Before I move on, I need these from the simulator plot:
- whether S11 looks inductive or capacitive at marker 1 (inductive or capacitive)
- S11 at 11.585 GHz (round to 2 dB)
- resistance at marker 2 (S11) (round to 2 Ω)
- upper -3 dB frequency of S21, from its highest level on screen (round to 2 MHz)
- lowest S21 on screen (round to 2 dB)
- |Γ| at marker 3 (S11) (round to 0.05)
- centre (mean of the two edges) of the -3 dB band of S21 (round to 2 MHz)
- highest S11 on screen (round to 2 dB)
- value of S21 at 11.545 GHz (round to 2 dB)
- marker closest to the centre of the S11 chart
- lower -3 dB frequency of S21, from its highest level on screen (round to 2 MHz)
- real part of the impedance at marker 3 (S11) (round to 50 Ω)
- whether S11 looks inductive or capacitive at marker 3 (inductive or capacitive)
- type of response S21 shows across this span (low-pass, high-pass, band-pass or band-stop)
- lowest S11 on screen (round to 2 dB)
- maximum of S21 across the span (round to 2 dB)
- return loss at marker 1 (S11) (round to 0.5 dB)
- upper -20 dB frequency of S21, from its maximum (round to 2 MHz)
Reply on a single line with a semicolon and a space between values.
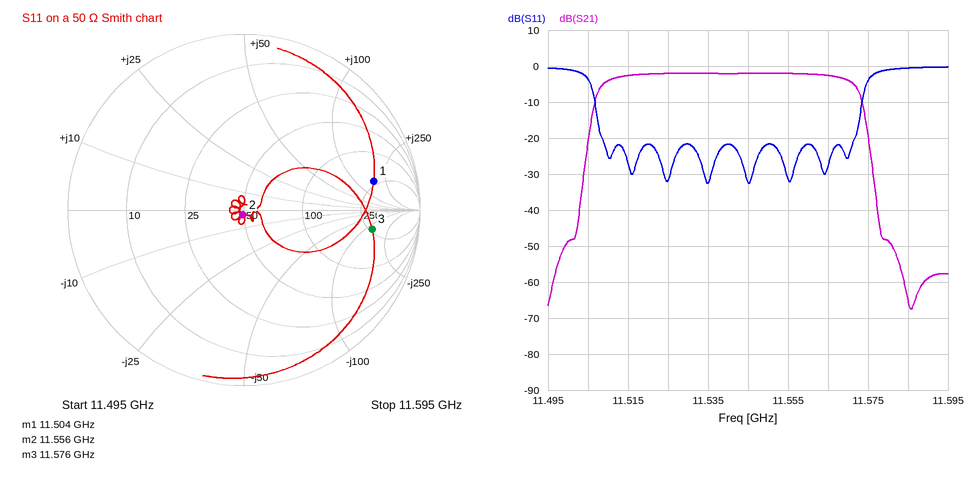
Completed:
inductive; 0 dB; 50 Ω; 11.572 GHz; -68 dB; 0.75; 11.540 GHz; 0 dB; -2 dB; marker 2; 11.508 GHz; 250 Ω; capacitive; band-pass; -32 dB; -2 dB; 2.5 dB; 11.576 GHz
